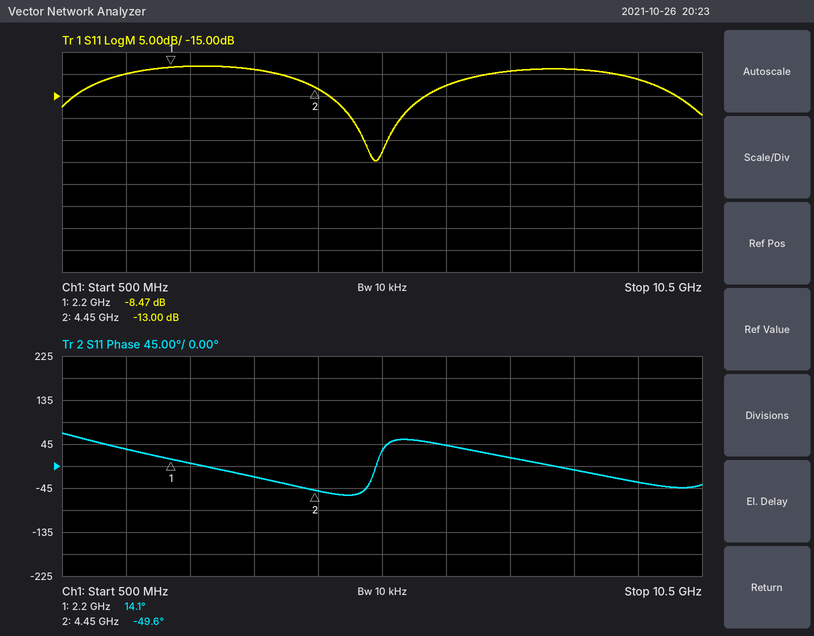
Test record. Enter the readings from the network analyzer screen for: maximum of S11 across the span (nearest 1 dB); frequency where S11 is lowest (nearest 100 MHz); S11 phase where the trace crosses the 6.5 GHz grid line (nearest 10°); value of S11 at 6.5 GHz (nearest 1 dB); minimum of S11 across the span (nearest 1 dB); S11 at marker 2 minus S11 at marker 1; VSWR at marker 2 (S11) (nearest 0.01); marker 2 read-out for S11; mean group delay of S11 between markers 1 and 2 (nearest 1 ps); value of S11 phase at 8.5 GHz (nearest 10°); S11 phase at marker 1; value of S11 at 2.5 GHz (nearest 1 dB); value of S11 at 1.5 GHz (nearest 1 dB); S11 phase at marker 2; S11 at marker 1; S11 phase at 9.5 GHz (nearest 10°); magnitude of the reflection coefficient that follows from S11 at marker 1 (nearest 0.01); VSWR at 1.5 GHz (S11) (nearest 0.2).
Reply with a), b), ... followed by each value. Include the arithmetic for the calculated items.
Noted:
a) -8 dB
b) 5.4 GHz
c) 40°
d) -13 dB
e) -30 dB
f) -13 − (-8.47) = -4.53 dB
g) (1 + 0.2239)/(1 − 0.2239) ≈ 1.58
h) -13.00 dB
i) −(-49.6° − (14.1°))/(360° × 2.25 GHz) ≈ 79 ps
j) -10°
k) 14.1°
l) -8 dB
m) -10 dB
n) -49.6°
o) -8.47 dB
p) -30°
q) 10^(-8.47/20) ≈ 0.38
r) |Γ| = 10^(-10/20) = 0.3162; VSWR = (1 + 0.3162)/(1 − 0.3162) ≈ 1.92, so 2.0 to the nearest 0.2
